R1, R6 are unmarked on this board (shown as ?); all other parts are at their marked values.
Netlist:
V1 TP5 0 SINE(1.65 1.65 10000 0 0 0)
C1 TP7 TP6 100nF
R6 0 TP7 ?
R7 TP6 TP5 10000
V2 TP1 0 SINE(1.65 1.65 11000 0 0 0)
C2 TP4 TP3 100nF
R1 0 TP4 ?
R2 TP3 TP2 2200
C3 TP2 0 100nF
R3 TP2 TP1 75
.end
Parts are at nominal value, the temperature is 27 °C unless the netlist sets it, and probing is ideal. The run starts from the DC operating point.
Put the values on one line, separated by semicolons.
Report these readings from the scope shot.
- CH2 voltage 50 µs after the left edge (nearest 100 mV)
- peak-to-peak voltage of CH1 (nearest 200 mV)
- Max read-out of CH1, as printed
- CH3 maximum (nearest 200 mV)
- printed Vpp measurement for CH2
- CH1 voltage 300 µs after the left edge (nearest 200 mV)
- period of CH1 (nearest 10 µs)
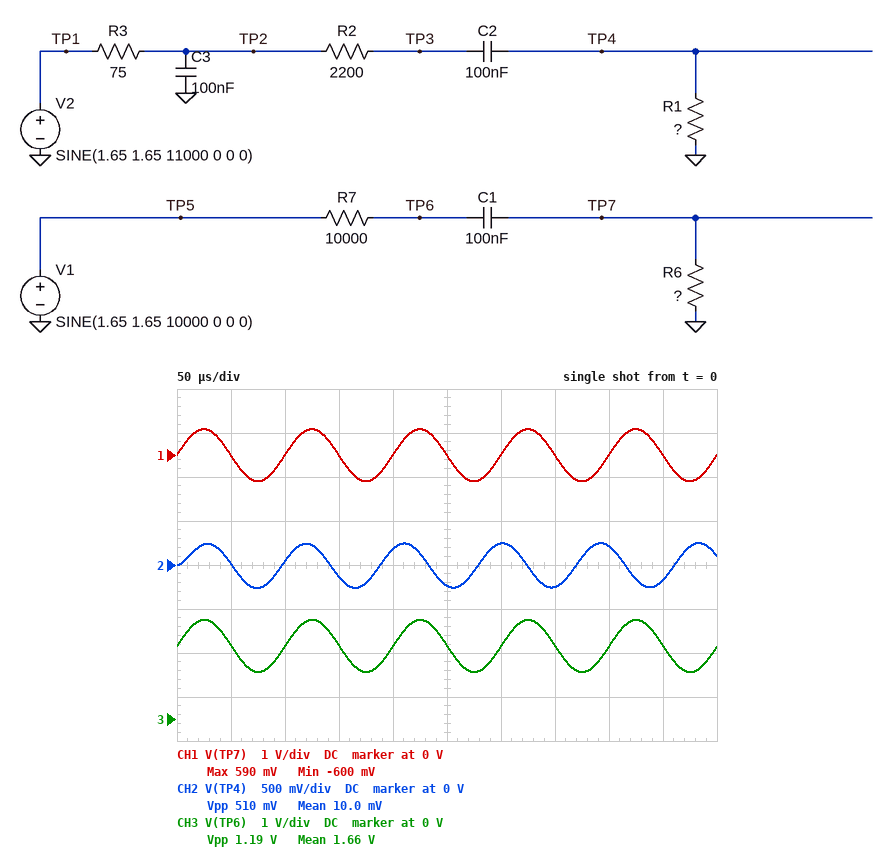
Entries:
0 V; 1.2 V; 590 mV; 2.2 V; 510 mV; 0 V; 100 µs
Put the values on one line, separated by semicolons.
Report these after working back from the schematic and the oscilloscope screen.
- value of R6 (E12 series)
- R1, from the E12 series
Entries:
5.6 kΩ; 470 Ω
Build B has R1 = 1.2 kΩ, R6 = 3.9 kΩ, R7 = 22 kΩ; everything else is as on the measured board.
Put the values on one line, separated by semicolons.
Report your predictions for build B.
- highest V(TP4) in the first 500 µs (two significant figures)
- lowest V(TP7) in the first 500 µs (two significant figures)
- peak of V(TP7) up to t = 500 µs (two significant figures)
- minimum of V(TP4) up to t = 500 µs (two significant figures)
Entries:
500 mV; -250 mV; 250 mV; -530 mV
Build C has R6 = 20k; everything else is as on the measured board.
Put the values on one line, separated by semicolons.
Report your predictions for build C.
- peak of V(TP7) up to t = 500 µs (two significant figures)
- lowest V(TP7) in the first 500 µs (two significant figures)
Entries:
1.1 V; -1.1 V
